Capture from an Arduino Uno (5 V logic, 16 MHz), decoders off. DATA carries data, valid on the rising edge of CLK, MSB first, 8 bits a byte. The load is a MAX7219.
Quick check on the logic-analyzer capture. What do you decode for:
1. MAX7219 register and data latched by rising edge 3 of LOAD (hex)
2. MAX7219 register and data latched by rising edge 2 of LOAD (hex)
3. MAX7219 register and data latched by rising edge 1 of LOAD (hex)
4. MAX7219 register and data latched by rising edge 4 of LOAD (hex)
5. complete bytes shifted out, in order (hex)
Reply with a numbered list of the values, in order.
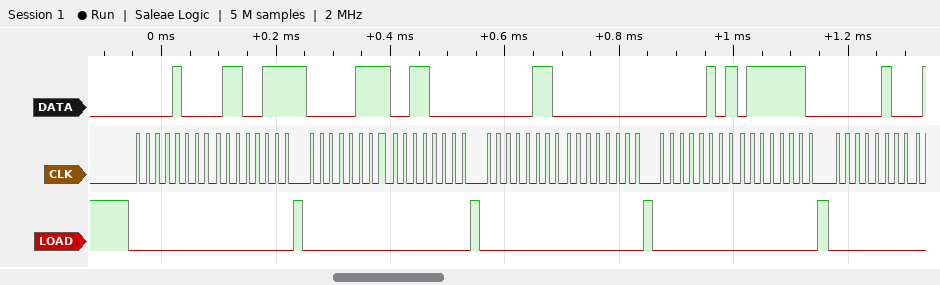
1. register 0x6, data 0x00
2. register 0x7, data 0x30
3. register 0x8, data 0x67
4. register 0x5, data 0x7E
5. 08 67 07 30 06 00 05 7E 04
